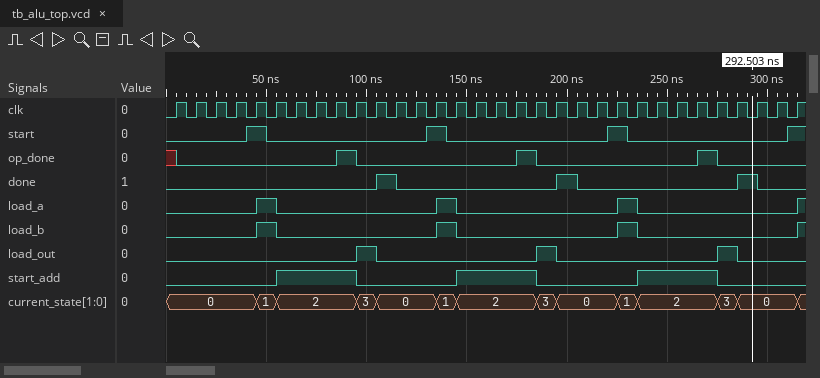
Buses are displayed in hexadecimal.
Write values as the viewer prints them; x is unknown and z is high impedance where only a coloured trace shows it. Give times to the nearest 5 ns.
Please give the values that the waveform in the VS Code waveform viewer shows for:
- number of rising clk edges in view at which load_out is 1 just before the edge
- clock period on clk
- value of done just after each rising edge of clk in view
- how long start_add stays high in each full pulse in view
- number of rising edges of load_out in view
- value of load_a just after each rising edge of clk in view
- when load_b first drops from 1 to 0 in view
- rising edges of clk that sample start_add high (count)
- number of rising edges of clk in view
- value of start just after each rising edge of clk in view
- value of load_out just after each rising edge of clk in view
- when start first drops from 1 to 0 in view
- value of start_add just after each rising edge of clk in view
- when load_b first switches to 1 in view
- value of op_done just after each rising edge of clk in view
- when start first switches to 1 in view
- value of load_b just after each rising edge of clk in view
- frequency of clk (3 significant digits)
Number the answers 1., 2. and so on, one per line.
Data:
1. 3
2. 10 ns
3. 0 0 0 0 0 0 0 0 0 0 1 0 0 0 0 0 0 0 0 1 0 0 0 0 0 0 0 0 1 0 0 0
4. 40 ns, 40 ns, 40 ns
5. 3
6. 0 0 0 0 1 0 0 0 0 0 0 0 0 1 0 0 0 0 0 0 0 0 1 0 0 0 0 0 0 0 0 1
7. 55 ns
8. 12
9. 32
10. 0 0 0 0 1 0 0 0 0 0 0 0 0 1 0 0 0 0 0 0 0 0 1 0 0 0 0 0 0 0 0 1
11. 0 0 0 0 0 0 0 0 0 1 0 0 0 0 0 0 0 0 1 0 0 0 0 0 0 0 0 1 0 0 0 0
12. 50 ns
13. 0 0 0 0 0 1 1 1 1 0 0 0 0 0 1 1 1 1 0 0 0 0 0 1 1 1 1 0 0 0 0 0
14. 45 ns
15. 0 0 0 0 0 0 0 0 1 0 0 0 0 0 0 0 0 1 0 0 0 0 0 0 0 0 1 0 0 0 0 0
16. 40 ns
17. 0 0 0 0 1 0 0 0 0 0 0 0 0 1 0 0 0 0 0 0 0 0 1 0 0 0 0 0 0 0 0 1
18. 100 MHz
